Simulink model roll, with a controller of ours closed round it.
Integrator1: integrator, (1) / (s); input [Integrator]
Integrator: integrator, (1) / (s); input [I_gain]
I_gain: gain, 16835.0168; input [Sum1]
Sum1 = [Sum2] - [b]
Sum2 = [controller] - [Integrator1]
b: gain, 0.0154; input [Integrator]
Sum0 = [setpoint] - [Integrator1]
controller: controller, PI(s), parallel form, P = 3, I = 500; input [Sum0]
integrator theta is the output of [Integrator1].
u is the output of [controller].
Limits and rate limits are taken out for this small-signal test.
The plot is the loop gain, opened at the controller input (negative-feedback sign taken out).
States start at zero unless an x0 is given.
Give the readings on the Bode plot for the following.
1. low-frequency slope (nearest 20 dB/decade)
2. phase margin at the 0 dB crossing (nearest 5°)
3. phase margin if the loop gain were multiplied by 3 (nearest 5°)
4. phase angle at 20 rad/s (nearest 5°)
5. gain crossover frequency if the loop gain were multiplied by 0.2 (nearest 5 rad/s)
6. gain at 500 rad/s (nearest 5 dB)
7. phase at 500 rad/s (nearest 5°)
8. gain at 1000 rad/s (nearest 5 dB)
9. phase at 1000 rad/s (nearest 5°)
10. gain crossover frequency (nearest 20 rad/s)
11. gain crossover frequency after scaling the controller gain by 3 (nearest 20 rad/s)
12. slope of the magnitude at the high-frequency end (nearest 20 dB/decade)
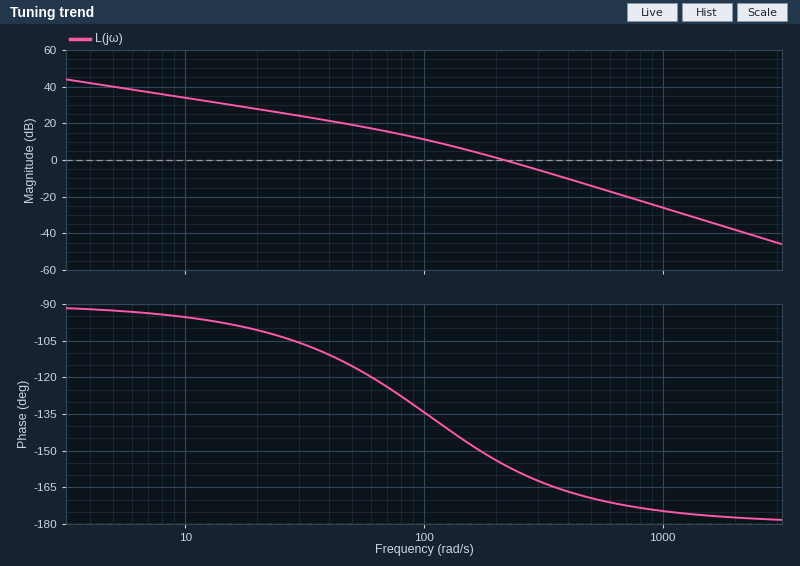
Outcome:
-20 dB/decade
25°
15°
-100°
80 rad/s
-15 dB
-170°
-25 dB
-175°
220 rad/s
380 rad/s
-40 dB/decade
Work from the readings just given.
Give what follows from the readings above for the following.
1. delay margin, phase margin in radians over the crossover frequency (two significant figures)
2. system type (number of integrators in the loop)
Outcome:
0.0020 s
1
